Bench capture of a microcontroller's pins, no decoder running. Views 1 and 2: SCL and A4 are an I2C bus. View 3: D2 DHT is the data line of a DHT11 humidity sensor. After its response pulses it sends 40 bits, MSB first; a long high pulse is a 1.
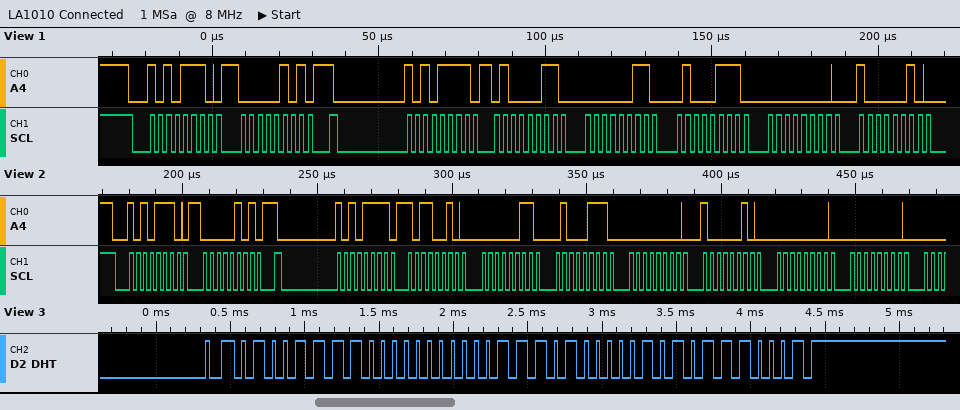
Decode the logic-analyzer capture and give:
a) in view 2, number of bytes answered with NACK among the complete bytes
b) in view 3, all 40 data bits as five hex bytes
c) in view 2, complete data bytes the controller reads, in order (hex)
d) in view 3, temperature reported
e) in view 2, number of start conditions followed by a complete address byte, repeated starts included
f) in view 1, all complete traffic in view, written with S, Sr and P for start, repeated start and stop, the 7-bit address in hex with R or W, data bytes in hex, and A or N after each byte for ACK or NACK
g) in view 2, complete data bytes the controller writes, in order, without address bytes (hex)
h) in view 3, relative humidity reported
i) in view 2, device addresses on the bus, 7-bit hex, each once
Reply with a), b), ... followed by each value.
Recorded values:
a) 0
b) 4F 00 1D 05 71
c) B2 03 47 00 82 00 00
d) 29.5 °C
e) 2
f) S 57W A 05 A Sr 57R A 43 A 03 A 47 A 00 A 82 A
g) 05
h) 79 %
i) 0x57
